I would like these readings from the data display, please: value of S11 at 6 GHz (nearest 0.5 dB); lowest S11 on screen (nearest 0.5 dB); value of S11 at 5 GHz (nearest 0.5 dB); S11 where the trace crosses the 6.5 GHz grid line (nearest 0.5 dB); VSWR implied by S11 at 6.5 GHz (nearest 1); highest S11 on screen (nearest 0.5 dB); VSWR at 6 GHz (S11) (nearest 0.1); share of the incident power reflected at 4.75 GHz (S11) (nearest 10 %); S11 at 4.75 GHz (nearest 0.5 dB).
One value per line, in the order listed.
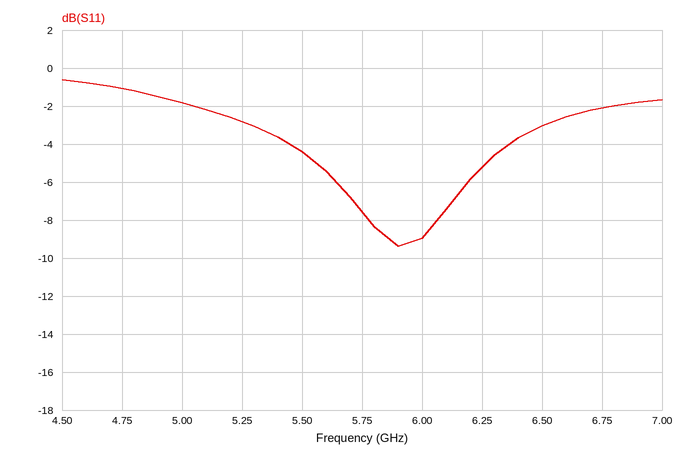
-9.0 dB
-9.5 dB
-2.0 dB
-3.0 dB
6
-0.5 dB
2.1
80 %
-1.0 dB
